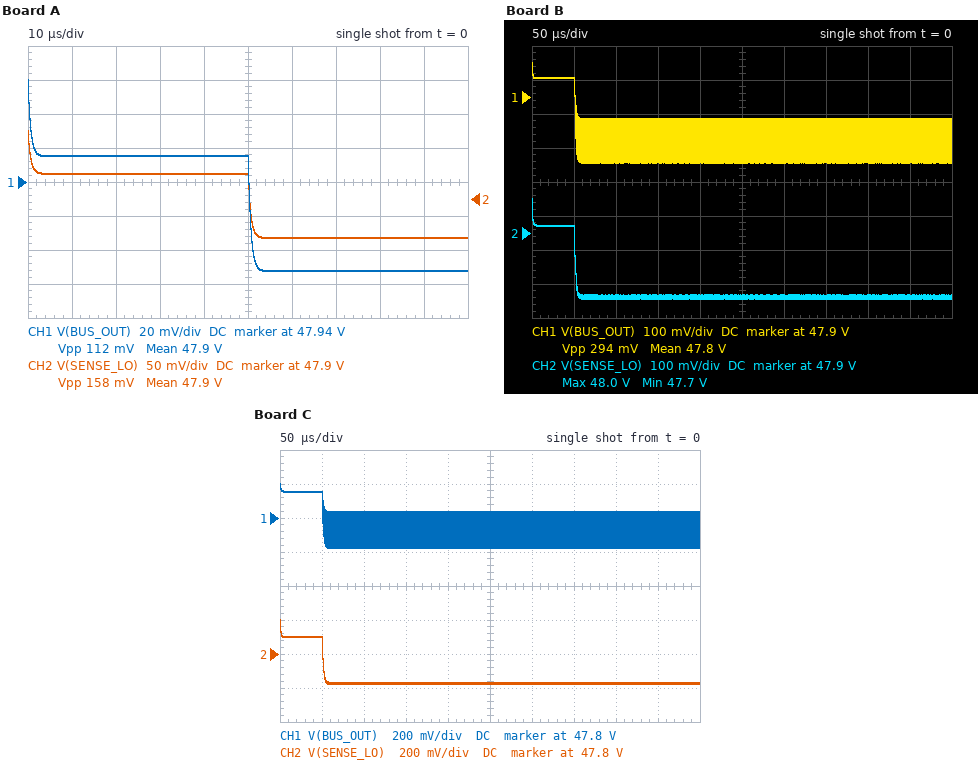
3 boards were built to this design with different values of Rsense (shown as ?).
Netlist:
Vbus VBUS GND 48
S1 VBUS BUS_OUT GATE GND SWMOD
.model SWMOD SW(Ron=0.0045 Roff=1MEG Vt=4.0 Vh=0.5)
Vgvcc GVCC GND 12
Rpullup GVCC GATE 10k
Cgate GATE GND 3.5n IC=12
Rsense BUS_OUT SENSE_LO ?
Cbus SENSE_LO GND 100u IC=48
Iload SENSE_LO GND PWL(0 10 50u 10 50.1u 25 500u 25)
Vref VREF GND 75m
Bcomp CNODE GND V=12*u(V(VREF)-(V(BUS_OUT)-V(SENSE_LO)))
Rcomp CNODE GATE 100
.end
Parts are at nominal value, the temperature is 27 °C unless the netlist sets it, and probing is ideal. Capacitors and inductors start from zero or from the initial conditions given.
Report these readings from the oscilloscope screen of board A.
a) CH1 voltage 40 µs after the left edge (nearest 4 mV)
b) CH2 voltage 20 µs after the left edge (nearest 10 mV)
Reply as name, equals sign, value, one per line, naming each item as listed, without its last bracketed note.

CH1 voltage 40 µs after the left edge = 47.956 V
CH2 voltage 20 µs after the left edge = 47.94 V
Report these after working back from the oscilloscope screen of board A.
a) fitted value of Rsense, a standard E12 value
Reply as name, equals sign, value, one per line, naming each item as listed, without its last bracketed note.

fitted value of Rsense, a standard E12 value = 1.8 mΩ
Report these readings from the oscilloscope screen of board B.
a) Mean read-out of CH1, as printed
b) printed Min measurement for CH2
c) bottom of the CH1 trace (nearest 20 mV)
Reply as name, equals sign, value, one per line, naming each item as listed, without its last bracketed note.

Mean read-out of CH1, as printed = 47.8 V
printed Min measurement for CH2 = 47.7 V
bottom of the CH1 trace = 47.70 V
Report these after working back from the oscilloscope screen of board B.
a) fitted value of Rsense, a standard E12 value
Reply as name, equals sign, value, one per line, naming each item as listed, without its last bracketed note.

fitted value of Rsense, a standard E12 value = 3.3 mΩ
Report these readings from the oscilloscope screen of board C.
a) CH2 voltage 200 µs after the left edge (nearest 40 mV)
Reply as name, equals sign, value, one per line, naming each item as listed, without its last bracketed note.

CH2 voltage 200 µs after the left edge = 47.64 V
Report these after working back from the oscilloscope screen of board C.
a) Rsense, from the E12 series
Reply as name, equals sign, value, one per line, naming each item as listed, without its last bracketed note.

Rsense, from the E12 series = 5.6 mΩ
